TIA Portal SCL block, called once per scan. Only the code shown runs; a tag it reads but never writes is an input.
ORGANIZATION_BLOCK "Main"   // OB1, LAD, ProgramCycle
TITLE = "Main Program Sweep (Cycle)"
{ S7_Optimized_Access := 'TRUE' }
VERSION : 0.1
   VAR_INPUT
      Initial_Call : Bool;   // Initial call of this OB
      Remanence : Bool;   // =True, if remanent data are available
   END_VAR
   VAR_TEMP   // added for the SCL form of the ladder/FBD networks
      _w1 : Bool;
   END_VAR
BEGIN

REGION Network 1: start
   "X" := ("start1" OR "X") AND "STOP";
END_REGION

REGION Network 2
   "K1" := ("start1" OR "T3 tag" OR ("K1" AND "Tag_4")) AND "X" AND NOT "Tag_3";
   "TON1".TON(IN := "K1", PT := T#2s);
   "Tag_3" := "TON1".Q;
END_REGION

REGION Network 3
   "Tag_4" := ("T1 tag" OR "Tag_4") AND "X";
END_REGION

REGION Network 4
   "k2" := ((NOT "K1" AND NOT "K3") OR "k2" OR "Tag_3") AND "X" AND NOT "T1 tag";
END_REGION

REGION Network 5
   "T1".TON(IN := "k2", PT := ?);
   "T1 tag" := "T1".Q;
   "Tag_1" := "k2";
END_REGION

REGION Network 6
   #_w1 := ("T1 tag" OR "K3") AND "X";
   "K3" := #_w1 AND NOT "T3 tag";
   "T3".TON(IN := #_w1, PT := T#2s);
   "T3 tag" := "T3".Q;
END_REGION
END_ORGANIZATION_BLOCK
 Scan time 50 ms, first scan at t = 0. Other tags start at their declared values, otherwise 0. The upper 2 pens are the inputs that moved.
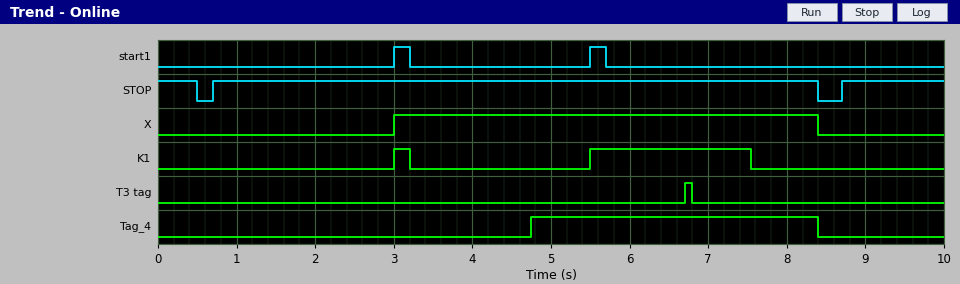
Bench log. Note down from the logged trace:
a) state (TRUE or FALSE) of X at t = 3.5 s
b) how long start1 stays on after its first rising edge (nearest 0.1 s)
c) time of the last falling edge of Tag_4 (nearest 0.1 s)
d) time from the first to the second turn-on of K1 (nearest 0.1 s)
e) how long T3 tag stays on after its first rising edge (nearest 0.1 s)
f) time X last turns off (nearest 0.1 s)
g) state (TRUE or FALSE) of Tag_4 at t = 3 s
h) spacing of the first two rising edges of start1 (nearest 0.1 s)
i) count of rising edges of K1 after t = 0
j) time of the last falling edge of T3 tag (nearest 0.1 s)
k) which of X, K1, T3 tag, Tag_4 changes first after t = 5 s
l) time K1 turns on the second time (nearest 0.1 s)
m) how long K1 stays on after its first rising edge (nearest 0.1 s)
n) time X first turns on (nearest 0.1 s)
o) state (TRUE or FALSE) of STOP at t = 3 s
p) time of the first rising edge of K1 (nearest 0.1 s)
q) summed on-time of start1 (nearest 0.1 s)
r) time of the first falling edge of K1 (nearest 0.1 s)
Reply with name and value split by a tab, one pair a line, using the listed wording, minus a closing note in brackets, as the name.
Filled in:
state (TRUE or FALSE) of X at t = 3.5 s	TRUE
how long start1 stays on after its first rising edge	0.2 s
time of the last falling edge of Tag_4	8.4 s
time from the first to the second turn-on of K1	2.5 s
how long T3 tag stays on after its first rising edge	0.1 s
time X last turns off	8.4 s
state (TRUE or FALSE) of Tag_4 at t = 3 s	FALSE
spacing of the first two rising edges of start1	2.5 s
count of rising edges of K1 after t = 0	2
time of the last falling edge of T3 tag	6.8 s
which of X, K1, T3 tag, Tag_4 changes first after t = 5 s	K1
time K1 turns on the second time	5.5 s
how long K1 stays on after its first rising edge	0.2 s
time X first turns on	3.0 s
state (TRUE or FALSE) of STOP at t = 3 s	TRUE
time of the first rising edge of K1	3.0 s
summed on-time of start1	0.4 s
time of the first falling edge of K1	3.2 s
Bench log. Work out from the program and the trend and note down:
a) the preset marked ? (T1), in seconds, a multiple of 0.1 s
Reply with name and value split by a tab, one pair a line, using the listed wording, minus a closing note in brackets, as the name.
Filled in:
the preset marked ? (T1), in seconds, a multiple of 0.1 s	1.5 s
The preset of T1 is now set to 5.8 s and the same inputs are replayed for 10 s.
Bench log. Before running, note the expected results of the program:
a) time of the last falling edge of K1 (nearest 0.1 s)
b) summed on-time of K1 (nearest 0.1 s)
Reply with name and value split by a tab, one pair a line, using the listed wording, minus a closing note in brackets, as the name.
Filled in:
time of the last falling edge of K1	5.7 s
summed on-time of K1	0.4 s
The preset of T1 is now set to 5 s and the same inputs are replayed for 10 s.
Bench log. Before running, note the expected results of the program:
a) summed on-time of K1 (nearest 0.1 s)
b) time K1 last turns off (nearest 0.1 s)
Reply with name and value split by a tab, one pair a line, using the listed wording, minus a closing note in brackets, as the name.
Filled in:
summed on-time of K1	0.4 s
time K1 last turns off	5.7 s
